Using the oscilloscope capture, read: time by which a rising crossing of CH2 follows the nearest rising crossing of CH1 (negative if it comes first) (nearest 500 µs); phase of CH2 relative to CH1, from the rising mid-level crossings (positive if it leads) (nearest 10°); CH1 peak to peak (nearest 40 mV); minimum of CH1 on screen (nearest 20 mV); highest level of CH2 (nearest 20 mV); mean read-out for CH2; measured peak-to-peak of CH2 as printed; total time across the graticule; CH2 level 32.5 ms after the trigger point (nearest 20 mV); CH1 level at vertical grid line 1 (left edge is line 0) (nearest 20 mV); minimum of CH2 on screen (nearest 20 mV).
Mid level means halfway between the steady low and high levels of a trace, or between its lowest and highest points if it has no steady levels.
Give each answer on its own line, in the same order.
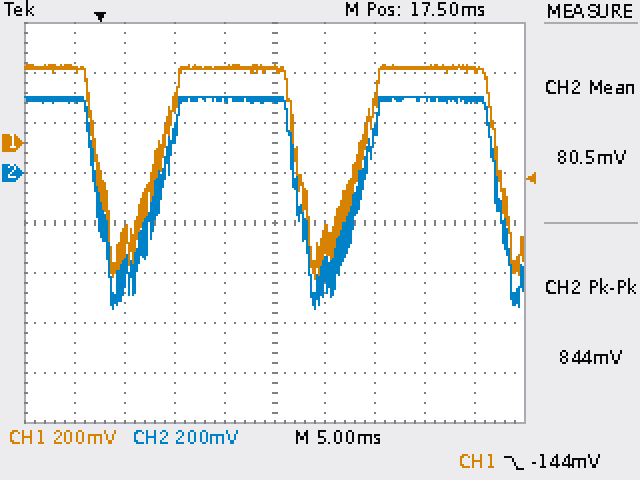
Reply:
0.0 ms
0°
840 mV
-540 mV
300 mV
80.5 mV
844 mV
50 ms
300 mV
300 mV
-540 mV
